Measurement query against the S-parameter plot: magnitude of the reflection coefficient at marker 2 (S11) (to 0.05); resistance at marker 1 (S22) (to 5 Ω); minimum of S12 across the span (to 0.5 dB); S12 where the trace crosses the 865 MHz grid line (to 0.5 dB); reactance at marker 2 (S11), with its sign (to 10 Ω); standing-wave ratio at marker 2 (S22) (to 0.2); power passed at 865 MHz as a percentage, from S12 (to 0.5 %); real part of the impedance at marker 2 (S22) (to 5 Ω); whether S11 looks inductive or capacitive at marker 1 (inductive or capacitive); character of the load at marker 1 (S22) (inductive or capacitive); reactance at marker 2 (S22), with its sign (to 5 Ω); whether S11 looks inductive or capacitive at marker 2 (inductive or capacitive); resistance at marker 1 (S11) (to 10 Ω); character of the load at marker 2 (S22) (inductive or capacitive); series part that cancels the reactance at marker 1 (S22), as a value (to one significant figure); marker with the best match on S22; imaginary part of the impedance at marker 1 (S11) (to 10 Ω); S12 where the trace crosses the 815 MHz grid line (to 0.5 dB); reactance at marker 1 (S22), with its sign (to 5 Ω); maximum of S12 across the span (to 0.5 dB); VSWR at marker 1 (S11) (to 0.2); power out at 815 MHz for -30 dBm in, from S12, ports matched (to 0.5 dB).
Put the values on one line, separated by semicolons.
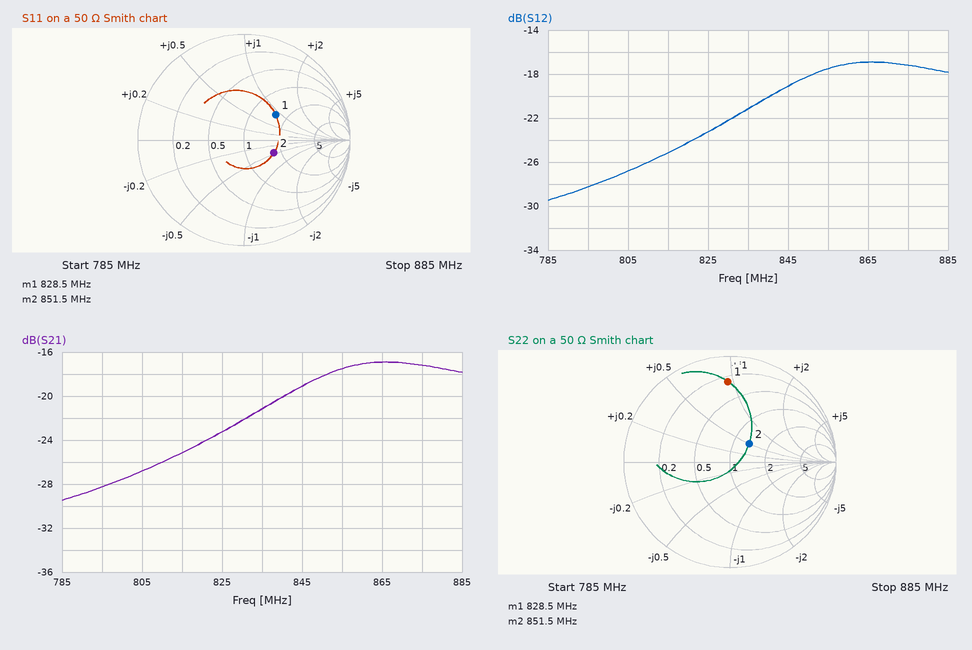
0.30; 15 Ω; -29.5 dB; -17.0 dB; -20 Ω; 1.6; 2.0 %; 65 Ω; inductive; inductive; +25 Ω; capacitive; 80 Ω; inductive; 4 pF; marker 2; +40 Ω; -25.0 dB; +45 Ω; -17.0 dB; 2.2; -55.0 dBm
